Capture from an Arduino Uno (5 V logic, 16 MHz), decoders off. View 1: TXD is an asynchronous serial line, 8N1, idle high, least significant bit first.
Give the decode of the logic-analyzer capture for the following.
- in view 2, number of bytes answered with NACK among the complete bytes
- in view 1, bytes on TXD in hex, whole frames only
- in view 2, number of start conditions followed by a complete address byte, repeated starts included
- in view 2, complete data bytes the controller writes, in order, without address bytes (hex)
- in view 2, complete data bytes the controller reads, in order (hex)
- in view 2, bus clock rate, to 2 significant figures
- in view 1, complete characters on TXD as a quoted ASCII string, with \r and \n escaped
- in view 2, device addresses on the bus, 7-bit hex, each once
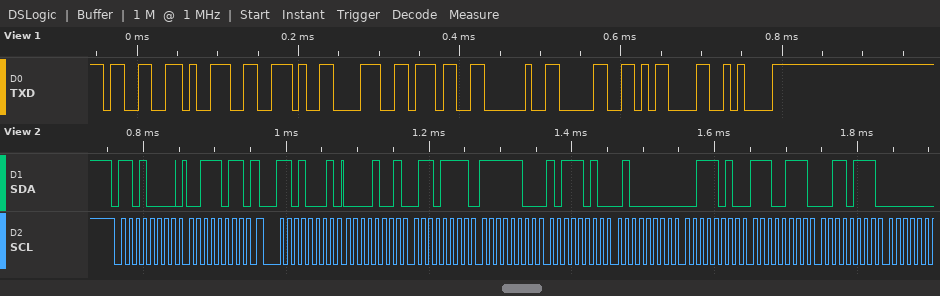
0
33 39 2E 38 37 20 30 0D 0A
2
3B
09 6F FC BA 40 3A E7 37
100 kHz
"39.87 0\r\n"
0x68
